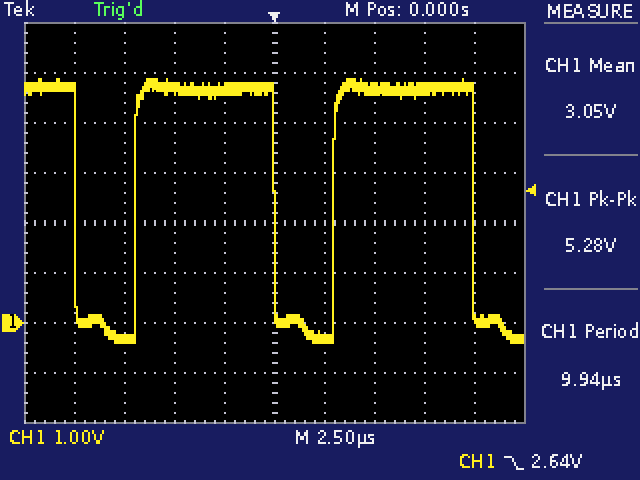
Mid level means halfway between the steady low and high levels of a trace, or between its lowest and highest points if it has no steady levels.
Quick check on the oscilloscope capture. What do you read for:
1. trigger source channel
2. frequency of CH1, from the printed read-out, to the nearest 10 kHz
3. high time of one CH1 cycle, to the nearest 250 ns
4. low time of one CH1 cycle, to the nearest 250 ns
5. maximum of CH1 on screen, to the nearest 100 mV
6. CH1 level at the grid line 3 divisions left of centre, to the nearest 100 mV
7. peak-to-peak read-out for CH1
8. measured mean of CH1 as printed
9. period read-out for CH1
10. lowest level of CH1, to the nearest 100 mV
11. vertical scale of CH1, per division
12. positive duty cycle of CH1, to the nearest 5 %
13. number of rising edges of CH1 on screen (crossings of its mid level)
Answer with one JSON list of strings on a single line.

["CH1", "100 kHz", "7.00 µs", "3.00 µs", "4.9 V", "-300 mV", "5.28 V", "3.05 V", "9.94 µs", "-400 mV", "1 V", "70 %", "2"]
